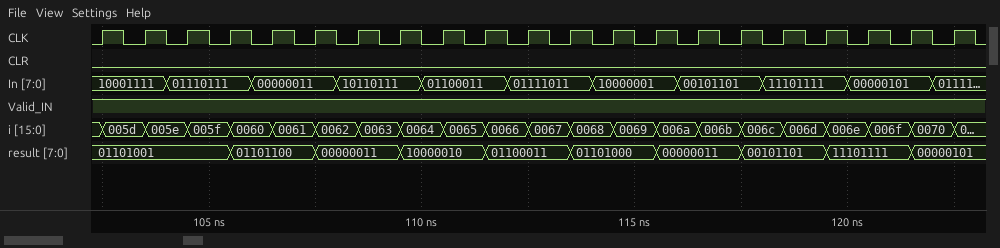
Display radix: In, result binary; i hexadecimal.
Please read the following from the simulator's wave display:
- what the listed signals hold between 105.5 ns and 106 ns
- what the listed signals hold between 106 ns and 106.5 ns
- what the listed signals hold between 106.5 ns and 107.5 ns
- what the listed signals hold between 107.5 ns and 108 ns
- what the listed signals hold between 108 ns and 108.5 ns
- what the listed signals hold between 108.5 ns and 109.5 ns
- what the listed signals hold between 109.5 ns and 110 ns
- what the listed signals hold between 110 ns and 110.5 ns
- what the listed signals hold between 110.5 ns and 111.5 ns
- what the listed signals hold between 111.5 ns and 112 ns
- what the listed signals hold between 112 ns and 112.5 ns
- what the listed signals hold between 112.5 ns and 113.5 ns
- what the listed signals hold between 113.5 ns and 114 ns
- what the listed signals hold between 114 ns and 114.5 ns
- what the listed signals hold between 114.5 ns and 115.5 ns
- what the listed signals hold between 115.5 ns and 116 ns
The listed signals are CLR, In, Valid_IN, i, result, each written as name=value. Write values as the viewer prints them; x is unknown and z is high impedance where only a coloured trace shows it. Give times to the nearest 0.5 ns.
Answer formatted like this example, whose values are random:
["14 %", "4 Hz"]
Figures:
["CLR=0, In=01110111, Valid_IN=1, i=0060, result=01101100", "CLR=0, In=00000011, Valid_IN=1, i=0060, result=01101100", "CLR=0, In=00000011, Valid_IN=1, i=0061, result=01101100", "CLR=0, In=00000011, Valid_IN=1, i=0062, result=00000011", "CLR=0, In=10110111, Valid_IN=1, i=0062, result=00000011", "CLR=0, In=10110111, Valid_IN=1, i=0063, result=00000011", "CLR=0, In=10110111, Valid_IN=1, i=0064, result=10000010", "CLR=0, In=01100011, Valid_IN=1, i=0064, result=10000010", "CLR=0, In=01100011, Valid_IN=1, i=0065, result=10000010", "CLR=0, In=01100011, Valid_IN=1, i=0066, result=01100011", "CLR=0, In=01111011, Valid_IN=1, i=0066, result=01100011", "CLR=0, In=01111011, Valid_IN=1, i=0067, result=01100011", "CLR=0, In=01111011, Valid_IN=1, i=0068, result=01101000", "CLR=0, In=10000001, Valid_IN=1, i=0068, result=01101000", "CLR=0, In=10000001, Valid_IN=1, i=0069, result=01101000", "CLR=0, In=10000001, Valid_IN=1, i=006a, result=00000011"]
